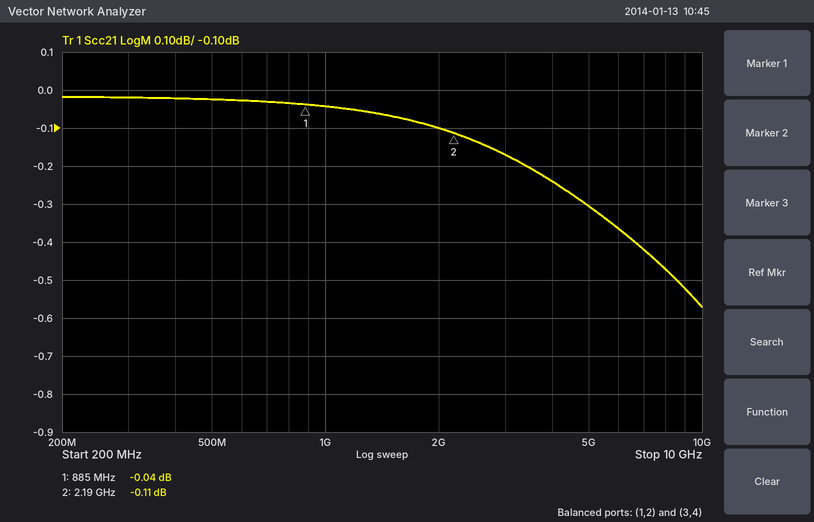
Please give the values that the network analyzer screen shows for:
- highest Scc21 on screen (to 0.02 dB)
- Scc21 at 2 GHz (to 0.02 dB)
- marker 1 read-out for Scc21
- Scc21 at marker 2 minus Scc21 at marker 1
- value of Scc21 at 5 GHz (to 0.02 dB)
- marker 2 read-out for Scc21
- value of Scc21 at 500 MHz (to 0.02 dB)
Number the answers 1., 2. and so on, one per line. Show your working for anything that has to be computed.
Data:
1. -0.02 dB
2. -0.10 dB
3. -0.04 dB
4. -0.11 − (-0.04) = -0.07 dB
5. -0.30 dB
6. -0.11 dB
7. -0.02 dB
